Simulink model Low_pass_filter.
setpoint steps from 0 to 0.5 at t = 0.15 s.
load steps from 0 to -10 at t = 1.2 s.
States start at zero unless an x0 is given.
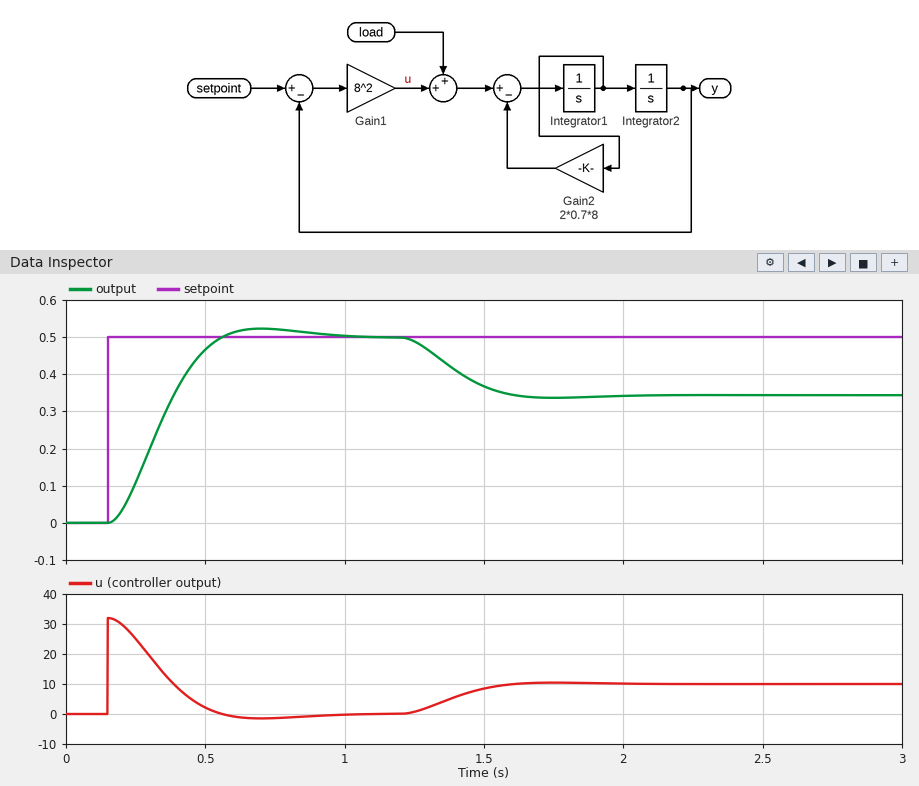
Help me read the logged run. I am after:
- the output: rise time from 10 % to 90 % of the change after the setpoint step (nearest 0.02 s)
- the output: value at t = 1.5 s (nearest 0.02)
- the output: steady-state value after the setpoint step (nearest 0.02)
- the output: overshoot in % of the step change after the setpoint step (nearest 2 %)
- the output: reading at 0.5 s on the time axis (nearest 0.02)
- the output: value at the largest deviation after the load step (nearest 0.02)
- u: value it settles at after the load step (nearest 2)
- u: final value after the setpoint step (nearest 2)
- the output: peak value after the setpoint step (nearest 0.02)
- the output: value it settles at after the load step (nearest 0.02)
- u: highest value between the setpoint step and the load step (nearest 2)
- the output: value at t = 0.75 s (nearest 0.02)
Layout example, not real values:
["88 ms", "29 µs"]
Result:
["0.26 s", "0.36", "0.50", "4 %", "0.46", "0.34", "10", "0", "0.52", "0.34", "32", "0.52"]
